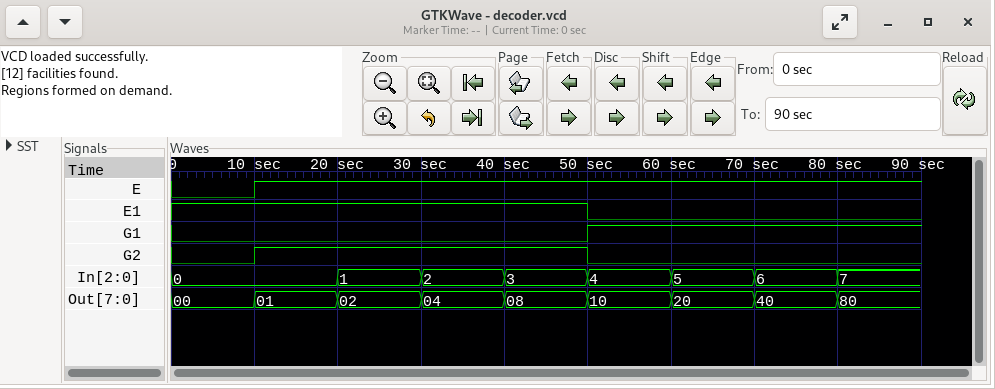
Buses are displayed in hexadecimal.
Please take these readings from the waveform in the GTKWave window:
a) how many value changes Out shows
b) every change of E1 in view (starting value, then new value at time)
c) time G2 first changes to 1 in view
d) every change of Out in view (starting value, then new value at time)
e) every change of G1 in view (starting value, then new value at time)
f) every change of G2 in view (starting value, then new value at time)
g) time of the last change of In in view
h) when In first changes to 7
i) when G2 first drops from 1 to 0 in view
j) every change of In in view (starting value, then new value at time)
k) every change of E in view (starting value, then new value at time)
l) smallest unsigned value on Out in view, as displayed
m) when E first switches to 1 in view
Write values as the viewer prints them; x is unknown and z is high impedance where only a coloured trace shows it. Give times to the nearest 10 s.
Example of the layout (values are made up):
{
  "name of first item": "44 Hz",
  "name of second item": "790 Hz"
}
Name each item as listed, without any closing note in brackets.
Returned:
{
  "how many value changes Out shows": "8",
  "every change of E1 in view": "1, 0 at 50 s",
  "time G2 first changes to 1 in view": "10 s",
  "every change of Out in view": "00, 01 at 10 s, 02 at 20 s, 04 at 30 s, 08 at 40 s, 10 at 50 s, 20 at 60 s, 40 at 70 s, 80 at 80 s",
  "every change of G1 in view": "0, 1 at 50 s",
  "every change of G2 in view": "0, 1 at 10 s, 0 at 50 s",
  "time of the last change of In in view": "80 s",
  "when In first changes to 7": "80 s",
  "when G2 first drops from 1 to 0 in view": "50 s",
  "every change of In in view": "0, 1 at 20 s, 2 at 30 s, 3 at 40 s, 4 at 50 s, 5 at 60 s, 6 at 70 s, 7 at 80 s",
  "every change of E in view": "0, 1 at 10 s",
  "smallest unsigned value on Out in view, as displayed": "00",
  "when E first switches to 1 in view": "10 s"
}
